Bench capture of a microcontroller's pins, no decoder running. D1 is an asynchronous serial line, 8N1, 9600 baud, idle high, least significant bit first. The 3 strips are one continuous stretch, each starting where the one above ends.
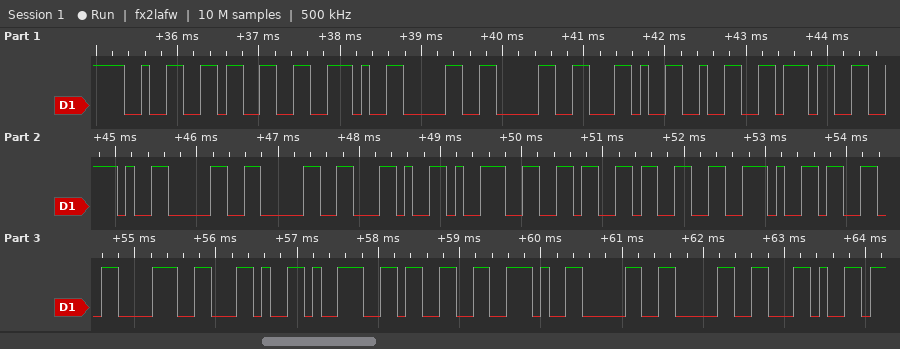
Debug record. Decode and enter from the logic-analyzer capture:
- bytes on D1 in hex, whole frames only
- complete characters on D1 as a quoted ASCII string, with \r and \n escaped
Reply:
32 33 2E 30 30 2C 32 37 2E 30 30 2C 39 36 33 2E 33 38 2C 39 33 2E 30 30 2C
"23.00,27.00,963.38,93.00,"
